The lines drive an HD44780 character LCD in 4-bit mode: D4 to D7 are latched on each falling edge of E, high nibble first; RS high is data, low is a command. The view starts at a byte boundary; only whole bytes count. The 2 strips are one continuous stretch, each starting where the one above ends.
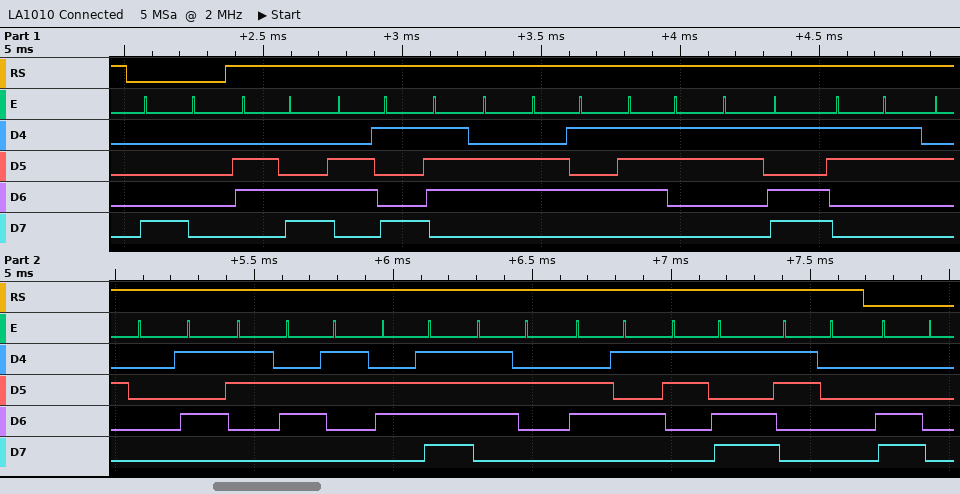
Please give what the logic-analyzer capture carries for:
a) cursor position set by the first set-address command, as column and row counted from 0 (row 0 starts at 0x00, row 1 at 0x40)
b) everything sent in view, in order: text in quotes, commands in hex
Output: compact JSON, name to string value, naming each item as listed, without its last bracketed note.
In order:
{"cursor position set by the first set-address command, as column and row counted from 0": "column 0, row 0", "everything sent in view, in order: text in quotes, commands in hex": "0x80 \"lives=3 Score=0\" 0xC0"}
